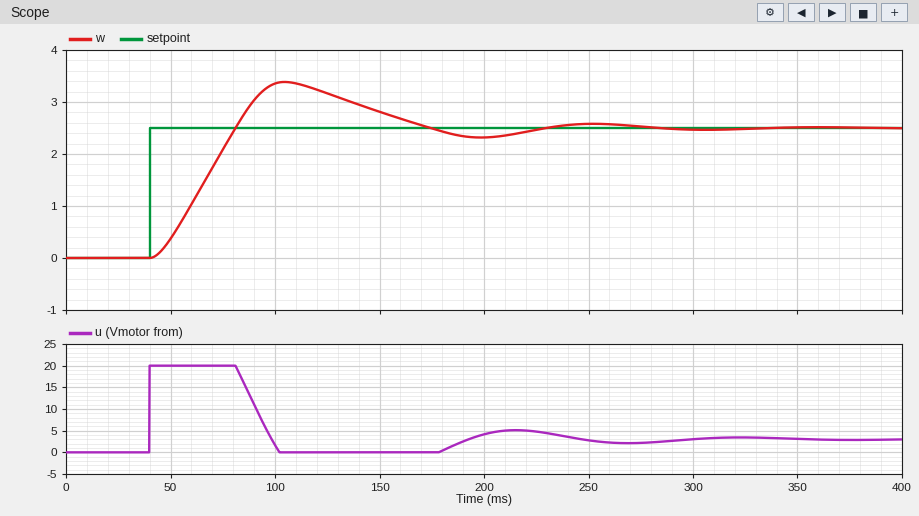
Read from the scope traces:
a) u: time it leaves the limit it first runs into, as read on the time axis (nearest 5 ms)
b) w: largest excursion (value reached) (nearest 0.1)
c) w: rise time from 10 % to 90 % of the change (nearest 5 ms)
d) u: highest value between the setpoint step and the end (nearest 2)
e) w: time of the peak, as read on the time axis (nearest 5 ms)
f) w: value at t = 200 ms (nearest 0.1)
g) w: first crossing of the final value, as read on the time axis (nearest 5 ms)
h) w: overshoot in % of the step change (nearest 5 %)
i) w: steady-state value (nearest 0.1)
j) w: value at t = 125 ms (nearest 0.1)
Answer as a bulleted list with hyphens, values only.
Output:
- 80 ms
- 3.4
- 30 ms
- 20
- 105 ms
- 2.3
- 80 ms
- 35 %
- 2.5
- 3.2
